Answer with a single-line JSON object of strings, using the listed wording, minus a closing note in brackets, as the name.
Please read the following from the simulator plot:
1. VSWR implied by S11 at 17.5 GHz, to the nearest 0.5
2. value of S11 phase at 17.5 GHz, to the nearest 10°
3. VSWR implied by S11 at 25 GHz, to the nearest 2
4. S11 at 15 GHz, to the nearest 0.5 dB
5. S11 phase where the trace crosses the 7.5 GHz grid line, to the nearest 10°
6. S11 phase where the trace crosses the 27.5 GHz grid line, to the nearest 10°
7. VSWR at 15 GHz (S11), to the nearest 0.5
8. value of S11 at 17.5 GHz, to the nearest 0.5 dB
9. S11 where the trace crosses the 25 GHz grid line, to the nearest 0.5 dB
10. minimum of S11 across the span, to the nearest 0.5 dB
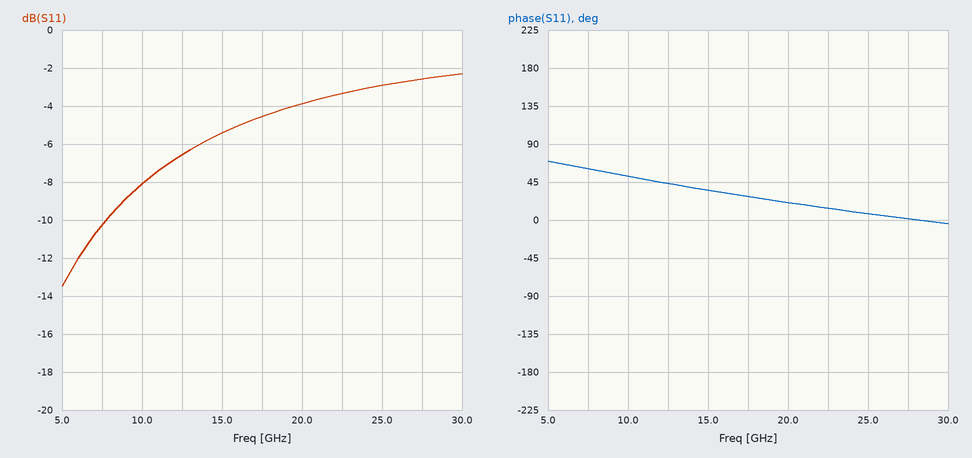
{"VSWR implied by S11 at 17.5 GHz, to the nearest 0.5": "4.0", "value of S11 phase at 17.5 GHz, to the nearest 10°": "30°", "VSWR implied by S11 at 25 GHz, to the nearest 2": "6", "S11 at 15 GHz, to the nearest 0.5 dB": "-5.5 dB", "S11 phase where the trace crosses the 7.5 GHz grid line, to the nearest 10°": "60°", "S11 phase where the trace crosses the 27.5 GHz grid line, to the nearest 10°": "0°", "VSWR at 15 GHz (S11), to the nearest 0.5": "3.5", "value of S11 at 17.5 GHz, to the nearest 0.5 dB": "-4.5 dB", "S11 where the trace crosses the 25 GHz grid line, to the nearest 0.5 dB": "-3.0 dB", "minimum of S11 across the span, to the nearest 0.5 dB": "-13.5 dB"}
